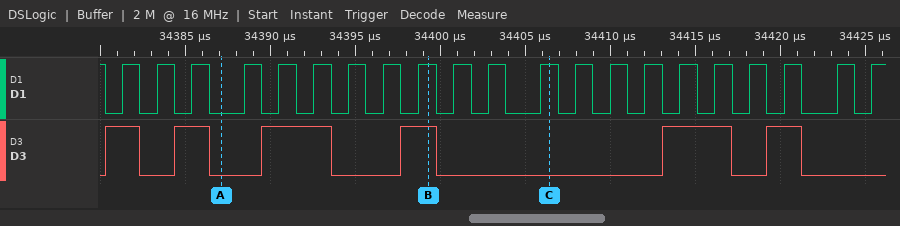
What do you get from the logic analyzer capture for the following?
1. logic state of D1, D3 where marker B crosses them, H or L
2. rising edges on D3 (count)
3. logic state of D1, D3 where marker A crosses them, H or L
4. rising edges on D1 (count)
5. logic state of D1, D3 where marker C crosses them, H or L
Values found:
D1=H, D3=H
6
D1=L, D3=L
21
D1=H, D3=L
